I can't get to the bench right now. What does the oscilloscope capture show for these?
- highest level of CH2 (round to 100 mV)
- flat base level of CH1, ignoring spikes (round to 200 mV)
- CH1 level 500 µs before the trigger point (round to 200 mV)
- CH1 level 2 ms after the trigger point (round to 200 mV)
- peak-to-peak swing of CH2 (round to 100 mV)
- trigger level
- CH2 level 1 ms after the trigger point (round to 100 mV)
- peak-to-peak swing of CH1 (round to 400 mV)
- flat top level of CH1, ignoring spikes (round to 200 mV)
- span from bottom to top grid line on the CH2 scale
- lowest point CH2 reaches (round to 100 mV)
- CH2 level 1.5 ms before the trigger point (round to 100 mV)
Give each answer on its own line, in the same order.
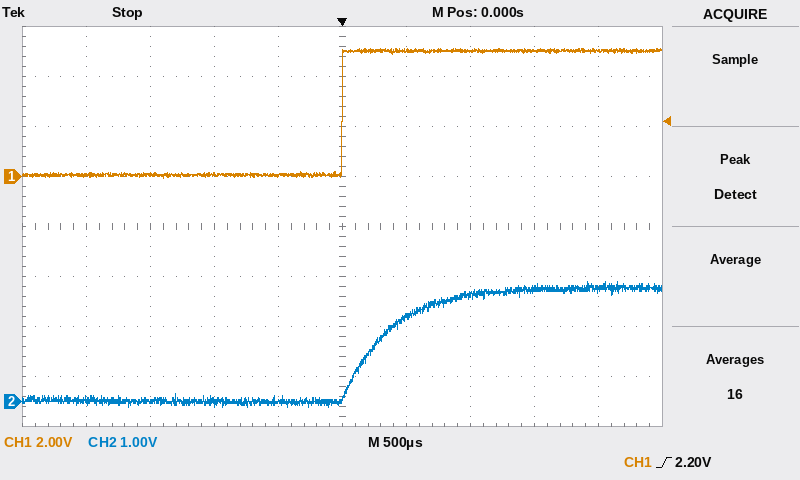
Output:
2.4 V
0.0 V
0.0 V
5.0 V
2.5 V
2.20 V
2.1 V
5.2 V
5.0 V
8 V
-100 mV
0.0 V
